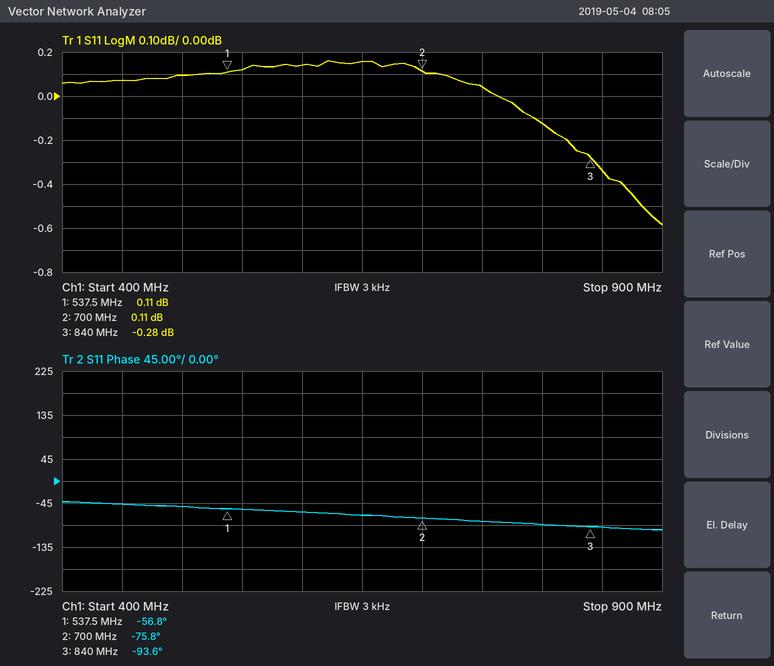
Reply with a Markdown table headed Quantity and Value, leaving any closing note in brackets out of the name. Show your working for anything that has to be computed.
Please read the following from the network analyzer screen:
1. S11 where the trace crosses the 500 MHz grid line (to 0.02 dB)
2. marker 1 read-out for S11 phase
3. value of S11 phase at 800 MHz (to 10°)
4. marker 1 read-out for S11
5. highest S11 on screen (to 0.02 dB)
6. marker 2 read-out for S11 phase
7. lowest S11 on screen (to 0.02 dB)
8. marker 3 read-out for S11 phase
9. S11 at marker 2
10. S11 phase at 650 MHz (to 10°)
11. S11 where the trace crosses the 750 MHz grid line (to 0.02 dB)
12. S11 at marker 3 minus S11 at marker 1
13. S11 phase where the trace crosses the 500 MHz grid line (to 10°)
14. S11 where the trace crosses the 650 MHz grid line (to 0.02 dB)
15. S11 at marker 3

| Quantity | Value |
|---|---|
| S11 where the trace crosses the 500 MHz grid line | 0.10 dB |
| marker 1 read-out for S11 phase | -56.8° |
| value of S11 phase at 800 MHz | -90° |
| marker 1 read-out for S11 | 0.11 dB |
| highest S11 on screen | 0.16 dB |
| marker 2 read-out for S11 phase | -75.8° |
| lowest S11 on screen | -0.58 dB |
| marker 3 read-out for S11 phase | -93.6° |
| S11 at marker 2 | 0.11 dB |
| S11 phase at 650 MHz | -70° |
| S11 where the trace crosses the 750 MHz grid line | 0.04 dB |
| S11 at marker 3 minus S11 at marker 1 | -0.28 − (0.11) = -0.39 dB |
| S11 phase where the trace crosses the 500 MHz grid line | -50° |
| S11 where the trace crosses the 650 MHz grid line | 0.16 dB |
| S11 at marker 3 | -0.28 dB |
